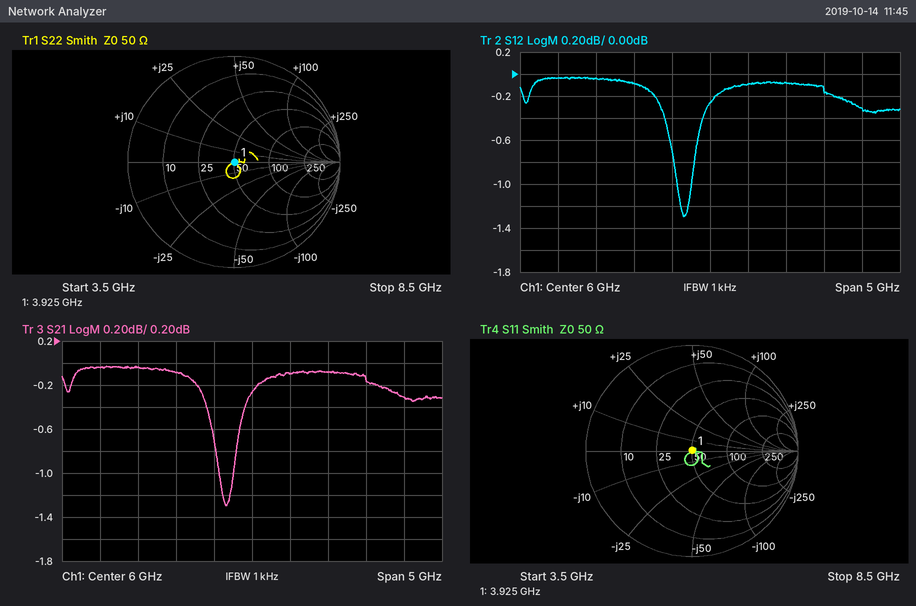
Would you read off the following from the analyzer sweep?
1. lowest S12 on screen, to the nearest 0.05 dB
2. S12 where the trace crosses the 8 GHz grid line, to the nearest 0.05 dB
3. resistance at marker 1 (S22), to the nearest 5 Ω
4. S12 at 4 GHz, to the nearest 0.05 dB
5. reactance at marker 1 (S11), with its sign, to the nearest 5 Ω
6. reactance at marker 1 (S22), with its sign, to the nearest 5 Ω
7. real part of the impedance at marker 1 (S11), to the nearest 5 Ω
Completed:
-1.30 dB
-0.30 dB
50 Ω
-0.05 dB
0 Ω
0 Ω
50 Ω
